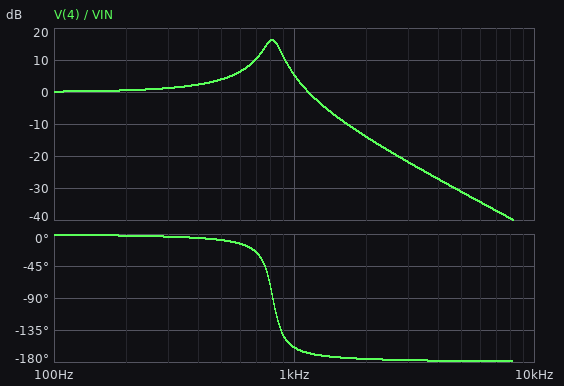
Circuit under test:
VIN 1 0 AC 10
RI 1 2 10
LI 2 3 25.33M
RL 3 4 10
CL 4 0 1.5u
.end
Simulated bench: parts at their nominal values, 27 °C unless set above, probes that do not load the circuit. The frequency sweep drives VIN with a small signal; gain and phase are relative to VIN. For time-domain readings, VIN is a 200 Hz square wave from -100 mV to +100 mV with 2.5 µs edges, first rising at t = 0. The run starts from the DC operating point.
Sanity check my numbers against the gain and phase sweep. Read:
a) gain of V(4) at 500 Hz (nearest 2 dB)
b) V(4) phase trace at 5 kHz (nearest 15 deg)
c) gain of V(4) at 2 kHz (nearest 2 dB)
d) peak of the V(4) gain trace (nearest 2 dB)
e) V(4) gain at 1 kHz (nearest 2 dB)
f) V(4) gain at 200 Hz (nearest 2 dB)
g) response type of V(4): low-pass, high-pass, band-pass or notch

4 dB
-180 deg
-14 dB
16 dB
6 dB
0 dB
low-pass
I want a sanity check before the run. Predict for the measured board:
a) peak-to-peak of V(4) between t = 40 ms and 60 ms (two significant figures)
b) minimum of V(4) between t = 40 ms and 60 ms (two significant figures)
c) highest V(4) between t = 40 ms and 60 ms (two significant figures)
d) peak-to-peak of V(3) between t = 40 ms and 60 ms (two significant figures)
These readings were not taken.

430 mV
-210 mV
210 mV
430 mV
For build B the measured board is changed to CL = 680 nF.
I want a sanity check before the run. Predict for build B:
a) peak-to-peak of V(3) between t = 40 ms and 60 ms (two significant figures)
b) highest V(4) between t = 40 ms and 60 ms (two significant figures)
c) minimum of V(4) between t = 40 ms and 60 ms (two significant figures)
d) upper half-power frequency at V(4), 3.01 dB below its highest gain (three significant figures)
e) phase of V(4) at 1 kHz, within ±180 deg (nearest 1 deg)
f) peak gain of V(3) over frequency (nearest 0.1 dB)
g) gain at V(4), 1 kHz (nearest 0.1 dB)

450 mV
220 mV
-220 mV
1.27 kHz
-15 deg
19.7 dB
9.6 dB
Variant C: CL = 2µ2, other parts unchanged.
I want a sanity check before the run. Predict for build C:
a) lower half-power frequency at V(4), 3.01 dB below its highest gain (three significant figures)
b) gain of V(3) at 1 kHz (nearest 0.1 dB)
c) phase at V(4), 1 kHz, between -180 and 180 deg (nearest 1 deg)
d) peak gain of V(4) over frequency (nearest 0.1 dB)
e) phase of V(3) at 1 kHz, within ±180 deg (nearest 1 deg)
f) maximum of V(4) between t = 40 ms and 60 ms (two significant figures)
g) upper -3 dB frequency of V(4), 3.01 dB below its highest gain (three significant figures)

602 Hz
-1.7 dB
-167 deg
14.6 dB
-159 deg
270 mV
729 Hz
